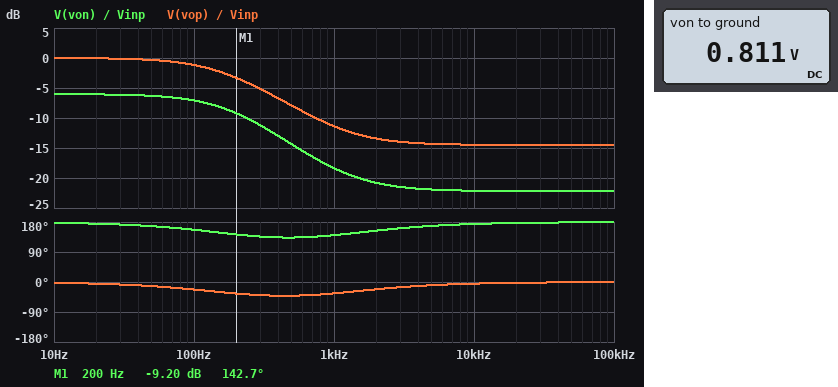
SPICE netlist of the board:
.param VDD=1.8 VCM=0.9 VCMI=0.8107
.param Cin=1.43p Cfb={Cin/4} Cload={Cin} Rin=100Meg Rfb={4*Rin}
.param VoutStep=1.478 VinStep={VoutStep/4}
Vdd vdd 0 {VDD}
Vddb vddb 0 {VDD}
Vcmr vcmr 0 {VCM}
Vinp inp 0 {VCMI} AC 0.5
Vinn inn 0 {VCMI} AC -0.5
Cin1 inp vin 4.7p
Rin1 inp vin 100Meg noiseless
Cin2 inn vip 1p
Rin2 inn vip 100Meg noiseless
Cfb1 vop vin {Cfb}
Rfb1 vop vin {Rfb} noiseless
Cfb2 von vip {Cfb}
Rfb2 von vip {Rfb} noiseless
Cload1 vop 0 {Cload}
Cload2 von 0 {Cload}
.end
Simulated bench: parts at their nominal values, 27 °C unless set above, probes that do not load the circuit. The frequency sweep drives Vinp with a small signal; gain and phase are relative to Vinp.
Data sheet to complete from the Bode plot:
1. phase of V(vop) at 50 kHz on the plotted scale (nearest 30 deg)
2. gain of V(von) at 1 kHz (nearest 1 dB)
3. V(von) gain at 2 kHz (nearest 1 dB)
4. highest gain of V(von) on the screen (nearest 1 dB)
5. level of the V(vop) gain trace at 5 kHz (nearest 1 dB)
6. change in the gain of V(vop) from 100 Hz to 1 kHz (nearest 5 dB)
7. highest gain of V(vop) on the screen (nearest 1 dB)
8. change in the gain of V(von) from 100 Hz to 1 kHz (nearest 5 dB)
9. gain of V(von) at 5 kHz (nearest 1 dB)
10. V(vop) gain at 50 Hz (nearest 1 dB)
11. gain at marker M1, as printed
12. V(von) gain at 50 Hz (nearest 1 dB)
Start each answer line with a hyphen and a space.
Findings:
- 0 deg
- -18 dB
- -21 dB
- -6 dB
- -14 dB
- -10 dB
- 0 dB
- -10 dB
- -22 dB
- 0 dB
- -9.20 dB
- -6 dB
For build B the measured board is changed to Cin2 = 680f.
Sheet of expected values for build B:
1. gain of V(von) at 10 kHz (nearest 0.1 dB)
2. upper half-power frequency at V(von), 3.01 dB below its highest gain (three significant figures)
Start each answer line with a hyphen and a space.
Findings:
- -22.9 dB
- 194 Hz
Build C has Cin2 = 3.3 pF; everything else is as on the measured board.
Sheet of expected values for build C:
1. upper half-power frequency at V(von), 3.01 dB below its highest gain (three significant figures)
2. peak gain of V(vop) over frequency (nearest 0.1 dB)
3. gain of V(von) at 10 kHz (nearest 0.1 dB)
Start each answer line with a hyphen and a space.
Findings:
- 187 Hz
- 0 dB
- -20.7 dB
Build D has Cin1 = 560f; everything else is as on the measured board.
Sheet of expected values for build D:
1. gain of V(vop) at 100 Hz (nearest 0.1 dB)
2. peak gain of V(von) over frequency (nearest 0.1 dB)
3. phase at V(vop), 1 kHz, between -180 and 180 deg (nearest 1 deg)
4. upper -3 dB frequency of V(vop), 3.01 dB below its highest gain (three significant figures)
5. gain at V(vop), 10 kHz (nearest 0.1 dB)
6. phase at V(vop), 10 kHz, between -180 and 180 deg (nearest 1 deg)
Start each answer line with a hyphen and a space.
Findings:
- -1.0 dB
- -6.0 dB
- -42 deg
- 194 Hz
- -17.4 dB
- -9 deg
